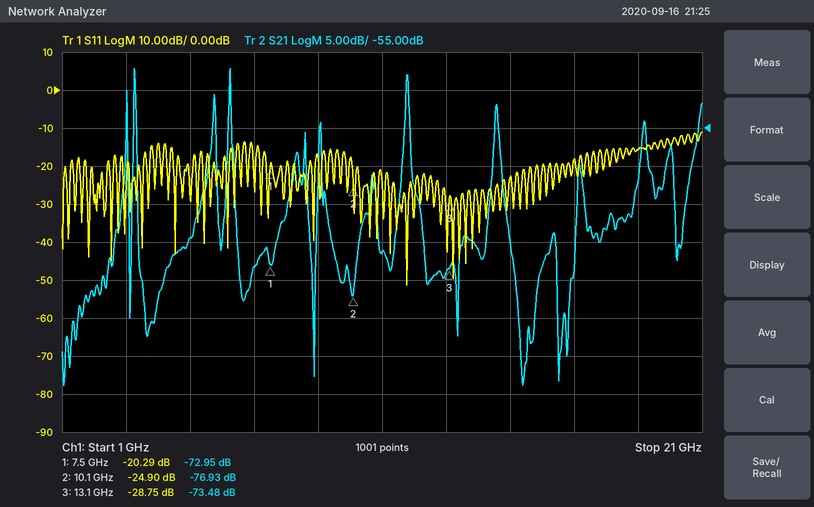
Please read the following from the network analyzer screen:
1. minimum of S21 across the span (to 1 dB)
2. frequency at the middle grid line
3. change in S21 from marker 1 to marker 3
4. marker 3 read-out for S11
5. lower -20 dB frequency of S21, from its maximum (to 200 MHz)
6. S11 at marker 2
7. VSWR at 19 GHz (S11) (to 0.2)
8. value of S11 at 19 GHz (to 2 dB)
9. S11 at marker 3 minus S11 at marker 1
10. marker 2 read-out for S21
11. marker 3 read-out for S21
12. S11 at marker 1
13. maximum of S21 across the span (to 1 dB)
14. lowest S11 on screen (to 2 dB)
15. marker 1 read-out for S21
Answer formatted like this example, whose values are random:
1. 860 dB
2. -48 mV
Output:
1. -89 dB
2. 11 GHz
3. -0.53 dB
4. -28.75 dB
5. 3.2 GHz
6. -24.90 dB
7. 1.4
8. -16 dB
9. -8.46 dB
10. -76.93 dB
11. -73.48 dB
12. -20.29 dB
13. -47 dB
14. -52 dB
15. -72.95 dB
